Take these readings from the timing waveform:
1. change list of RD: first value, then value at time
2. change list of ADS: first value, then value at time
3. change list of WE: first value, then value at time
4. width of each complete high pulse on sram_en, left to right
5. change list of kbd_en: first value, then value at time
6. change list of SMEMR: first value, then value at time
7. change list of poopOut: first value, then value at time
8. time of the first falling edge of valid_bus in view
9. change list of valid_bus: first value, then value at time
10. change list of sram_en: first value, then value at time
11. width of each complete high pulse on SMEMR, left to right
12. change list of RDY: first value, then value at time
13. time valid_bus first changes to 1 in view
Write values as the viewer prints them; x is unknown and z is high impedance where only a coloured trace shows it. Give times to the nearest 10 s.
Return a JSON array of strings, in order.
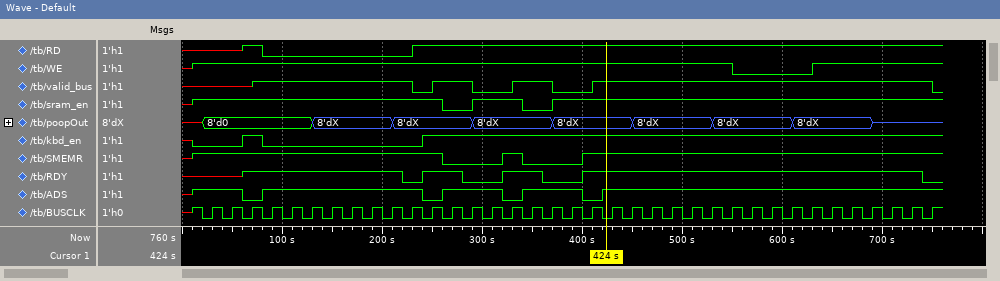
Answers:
["x, 1 at 60 s, 0 at 80 s, 1 at 230 s", "x, 1 at 10 s, 0 at 60 s, 1 at 80 s, 0 at 240 s, 1 at 260 s, 0 at 320 s, 1 at 340 s, 0 at 400 s, 1 at 420 s", "x, 1 at 10 s, 0 at 550 s, 1 at 630 s", "50 s", "x, 0 at 10 s, 1 at 60 s, 0 at 80 s, 1 at 240 s", "x, 1 at 10 s, 0 at 260 s, 1 at 320 s, 0 at 340 s, 1 at 400 s", "x, 8'd0 at 20 s, 8'dX at 130 s, 8'dX at 210 s, 8'dX at 290 s, 8'dX at 370 s, 8'dX at 450 s, 8'dX at 530 s, 8'dX at 610 s, z at 690 s", "230 s", "x, 1 at 70 s, 0 at 230 s, 1 at 250 s, 0 at 290 s, 1 at 330 s, 0 at 370 s, 1 at 410 s, 0 at 750 s", "x, 1 at 10 s, 0 at 260 s, 1 at 290 s, 0 at 340 s, 1 at 370 s", "20 s", "x, 1 at 60 s, 0 at 220 s, 1 at 240 s, 0 at 280 s, 1 at 320 s, 0 at 360 s, 1 at 400 s, 0 at 740 s", "70 s"]
